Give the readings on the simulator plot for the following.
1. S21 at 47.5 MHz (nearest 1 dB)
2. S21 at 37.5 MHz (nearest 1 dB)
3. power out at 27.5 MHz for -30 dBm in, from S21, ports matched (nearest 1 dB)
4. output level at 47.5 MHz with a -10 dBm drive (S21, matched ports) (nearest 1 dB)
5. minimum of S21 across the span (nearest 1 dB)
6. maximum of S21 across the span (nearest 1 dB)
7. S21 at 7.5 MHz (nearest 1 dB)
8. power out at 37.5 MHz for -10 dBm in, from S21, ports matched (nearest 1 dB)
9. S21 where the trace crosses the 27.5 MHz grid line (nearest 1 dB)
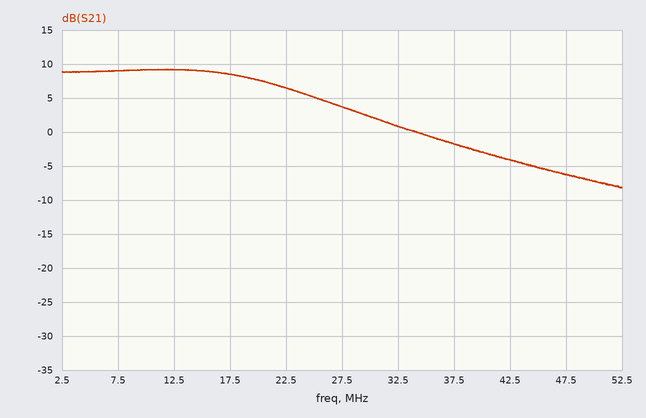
-6 dB
-2 dB
-26 dBm
-16 dBm
-8 dB
9 dB
9 dB
-12 dBm
4 dB
